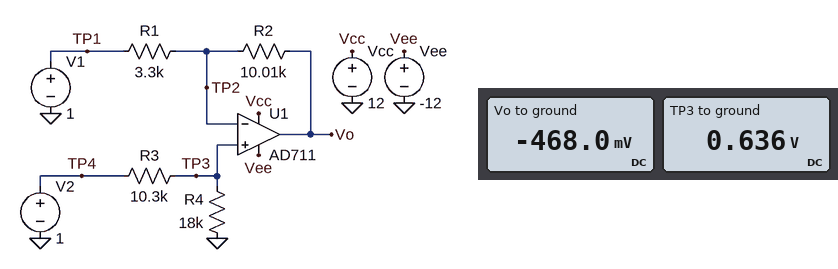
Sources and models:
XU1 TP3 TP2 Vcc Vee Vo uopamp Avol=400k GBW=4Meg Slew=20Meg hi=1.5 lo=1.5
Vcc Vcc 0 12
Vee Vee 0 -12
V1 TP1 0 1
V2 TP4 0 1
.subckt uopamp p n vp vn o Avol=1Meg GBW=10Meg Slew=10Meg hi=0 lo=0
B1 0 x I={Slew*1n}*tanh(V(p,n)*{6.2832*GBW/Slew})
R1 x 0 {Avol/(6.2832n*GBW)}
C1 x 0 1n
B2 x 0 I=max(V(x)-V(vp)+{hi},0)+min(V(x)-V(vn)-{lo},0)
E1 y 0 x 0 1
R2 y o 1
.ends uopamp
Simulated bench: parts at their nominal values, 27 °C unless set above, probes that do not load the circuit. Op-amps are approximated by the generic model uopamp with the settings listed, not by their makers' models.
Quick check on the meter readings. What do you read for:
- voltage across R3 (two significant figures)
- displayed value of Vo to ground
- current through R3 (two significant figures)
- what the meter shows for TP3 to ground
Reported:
360 mV
-468.0 mV
35 µA
0.636 V
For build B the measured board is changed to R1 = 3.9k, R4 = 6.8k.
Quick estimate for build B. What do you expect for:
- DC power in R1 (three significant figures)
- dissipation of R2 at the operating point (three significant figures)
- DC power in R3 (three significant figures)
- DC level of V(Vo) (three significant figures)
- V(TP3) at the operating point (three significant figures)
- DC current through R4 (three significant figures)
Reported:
93.0 µW
239 µW
35.2 µW
-1.15 V
398 mV
58.5 µA
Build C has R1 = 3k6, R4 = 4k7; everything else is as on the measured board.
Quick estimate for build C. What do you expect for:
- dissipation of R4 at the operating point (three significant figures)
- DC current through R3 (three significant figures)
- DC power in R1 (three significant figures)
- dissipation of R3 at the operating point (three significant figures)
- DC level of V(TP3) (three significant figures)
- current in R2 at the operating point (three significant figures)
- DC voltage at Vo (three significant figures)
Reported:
20.9 µW
66.7 µA
131 µW
45.8 µW
313 mV
191 µA
-1.60 V
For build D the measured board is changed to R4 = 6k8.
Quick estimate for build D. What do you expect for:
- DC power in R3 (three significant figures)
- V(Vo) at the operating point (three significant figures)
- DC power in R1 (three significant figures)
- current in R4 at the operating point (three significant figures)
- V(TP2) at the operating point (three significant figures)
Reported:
35.2 µW
-1.43 V
110 µW
58.5 µA
398 mV
